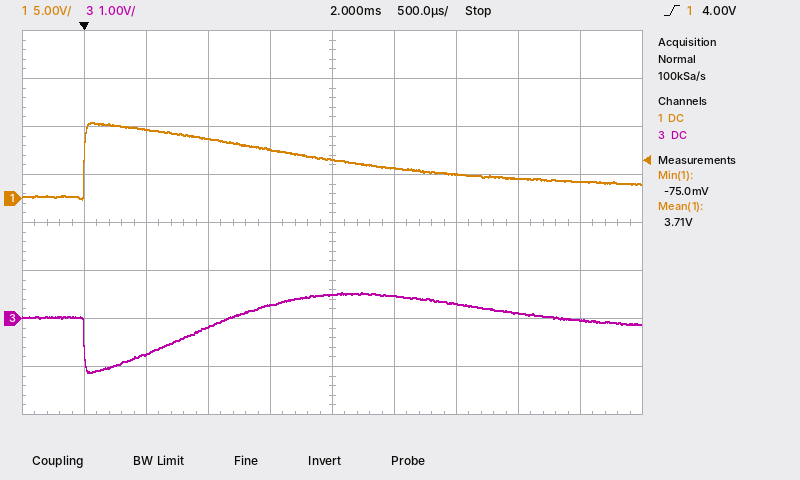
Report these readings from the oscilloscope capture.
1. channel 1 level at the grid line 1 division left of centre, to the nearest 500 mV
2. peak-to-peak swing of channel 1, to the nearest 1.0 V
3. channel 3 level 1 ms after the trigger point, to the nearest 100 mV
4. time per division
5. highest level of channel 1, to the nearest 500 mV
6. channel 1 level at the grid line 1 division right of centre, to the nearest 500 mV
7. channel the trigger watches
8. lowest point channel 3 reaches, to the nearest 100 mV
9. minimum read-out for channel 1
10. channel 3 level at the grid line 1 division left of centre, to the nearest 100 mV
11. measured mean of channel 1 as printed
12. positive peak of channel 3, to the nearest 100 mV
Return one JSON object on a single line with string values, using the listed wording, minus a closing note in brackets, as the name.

{"channel 1 level at the grid line 1 division left of centre, to the nearest 500 mV": "5.0 V", "peak-to-peak swing of channel 1, to the nearest 1.0 V": "8.0 V", "channel 3 level 1 ms after the trigger point, to the nearest 100 mV": "-200 mV", "time per division": "500 µs", "highest level of channel 1, to the nearest 500 mV": "8.0 V", "channel 1 level at the grid line 1 division right of centre, to the nearest 500 mV": "3.0 V", "channel the trigger watches": "channel 1", "lowest point channel 3 reaches, to the nearest 100 mV": "-1.1 V", "minimum read-out for channel 1": "-75.0 mV", "channel 3 level at the grid line 1 division left of centre, to the nearest 100 mV": "300 mV", "measured mean of channel 1 as printed": "3.71 V", "positive peak of channel 3, to the nearest 100 mV": "500 mV"}
